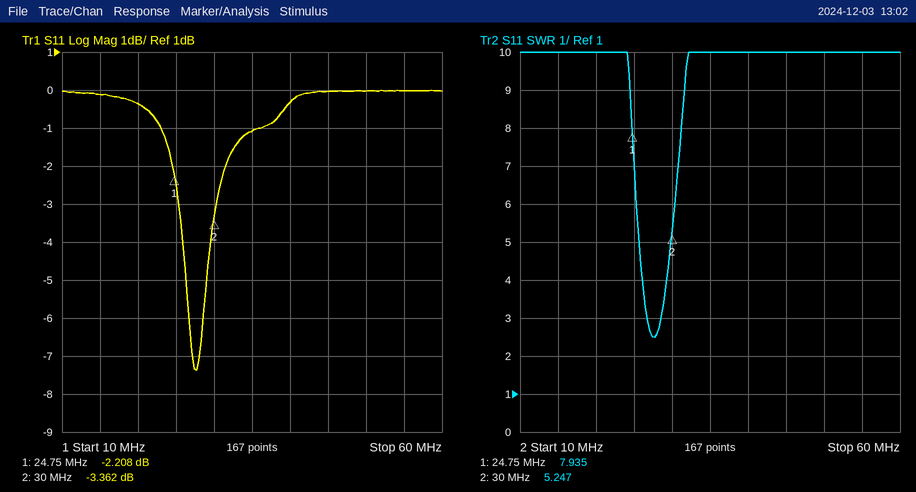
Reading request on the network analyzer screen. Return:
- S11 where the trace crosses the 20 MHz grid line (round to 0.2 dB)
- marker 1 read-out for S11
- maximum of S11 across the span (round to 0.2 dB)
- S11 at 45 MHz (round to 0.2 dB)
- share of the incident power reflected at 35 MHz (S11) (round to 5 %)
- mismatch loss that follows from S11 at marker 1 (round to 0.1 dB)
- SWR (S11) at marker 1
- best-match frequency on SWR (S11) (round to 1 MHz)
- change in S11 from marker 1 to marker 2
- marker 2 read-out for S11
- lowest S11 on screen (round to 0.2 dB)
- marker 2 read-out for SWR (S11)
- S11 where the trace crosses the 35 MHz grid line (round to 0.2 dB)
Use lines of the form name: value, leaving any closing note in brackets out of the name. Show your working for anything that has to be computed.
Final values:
S11 where the trace crosses the 20 MHz grid line: -0.4 dB
marker 1 read-out for S11: -2.208 dB
maximum of S11 across the span: 0.0 dB
S11 at 45 MHz: 0.0 dB
share of the incident power reflected at 35 MHz (S11): 10^(-1/10) ≈ 79.4 %, so 80 % to the nearest 5 %
mismatch loss that follows from S11 at marker 1: −10 log10(1 − 10^(-2.208/10)) ≈ 4.0 dB
SWR (S11) at marker 1: 7.935
best-match frequency on SWR (S11): 28 MHz
change in S11 from marker 1 to marker 2: -3.362 − (-2.208) = -1.154 dB
marker 2 read-out for S11: -3.362 dB
lowest S11 on screen: -7.4 dB
marker 2 read-out for SWR: 5.247
S11 where the trace crosses the 35 MHz grid line: -1.0 dB
